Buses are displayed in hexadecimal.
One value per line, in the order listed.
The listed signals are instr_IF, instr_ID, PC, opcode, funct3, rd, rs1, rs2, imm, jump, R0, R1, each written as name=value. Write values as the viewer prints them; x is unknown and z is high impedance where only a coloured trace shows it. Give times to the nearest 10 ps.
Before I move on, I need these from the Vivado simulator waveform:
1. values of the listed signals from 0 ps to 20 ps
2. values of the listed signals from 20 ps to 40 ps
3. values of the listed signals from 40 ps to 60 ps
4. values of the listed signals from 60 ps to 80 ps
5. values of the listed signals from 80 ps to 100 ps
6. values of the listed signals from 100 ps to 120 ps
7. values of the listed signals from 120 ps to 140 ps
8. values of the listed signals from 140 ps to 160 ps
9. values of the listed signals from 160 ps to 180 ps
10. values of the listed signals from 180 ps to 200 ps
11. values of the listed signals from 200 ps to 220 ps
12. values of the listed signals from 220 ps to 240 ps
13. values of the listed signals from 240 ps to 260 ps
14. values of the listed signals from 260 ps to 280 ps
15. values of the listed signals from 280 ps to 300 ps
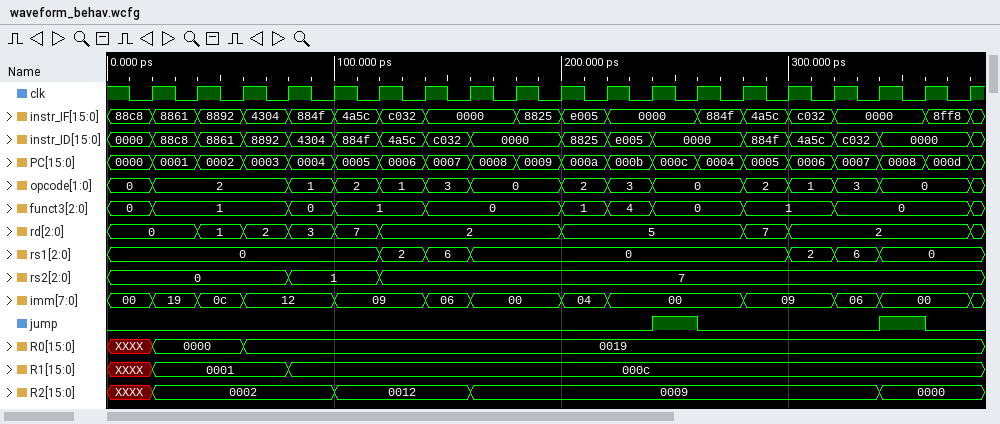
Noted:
instr_IF=88c8, instr_ID=0000, PC=0000, opcode=0, funct3=0, rd=0, rs1=0, rs2=0, imm=00, jump=0, R0=XXXX, R1=XXXX
instr_IF=8861, instr_ID=88c8, PC=0001, opcode=2, funct3=1, rd=0, rs1=0, rs2=0, imm=19, jump=0, R0=0000, R1=0001
instr_IF=8892, instr_ID=8861, PC=0002, opcode=2, funct3=1, rd=1, rs1=0, rs2=0, imm=0c, jump=0, R0=0000, R1=0001
instr_IF=4304, instr_ID=8892, PC=0003, opcode=2, funct3=1, rd=2, rs1=0, rs2=0, imm=12, jump=0, R0=0019, R1=0001
instr_IF=884f, instr_ID=4304, PC=0004, opcode=1, funct3=0, rd=3, rs1=0, rs2=1, imm=12, jump=0, R0=0019, R1=000c
instr_IF=4a5c, instr_ID=884f, PC=0005, opcode=2, funct3=1, rd=7, rs1=0, rs2=1, imm=09, jump=0, R0=0019, R1=000c
instr_IF=c032, instr_ID=4a5c, PC=0006, opcode=1, funct3=1, rd=2, rs1=2, rs2=7, imm=09, jump=0, R0=0019, R1=000c
instr_IF=0000, instr_ID=c032, PC=0007, opcode=3, funct3=0, rd=2, rs1=6, rs2=7, imm=06, jump=0, R0=0019, R1=000c
instr_IF=0000, instr_ID=0000, PC=0008, opcode=0, funct3=0, rd=2, rs1=0, rs2=7, imm=00, jump=0, R0=0019, R1=000c
instr_IF=8825, instr_ID=0000, PC=0009, opcode=0, funct3=0, rd=2, rs1=0, rs2=7, imm=00, jump=0, R0=0019, R1=000c
instr_IF=e005, instr_ID=8825, PC=000a, opcode=2, funct3=1, rd=5, rs1=0, rs2=7, imm=04, jump=0, R0=0019, R1=000c
instr_IF=0000, instr_ID=e005, PC=000b, opcode=3, funct3=4, rd=5, rs1=0, rs2=7, imm=00, jump=0, R0=0019, R1=000c
instr_IF=0000, instr_ID=0000, PC=000c, opcode=0, funct3=0, rd=5, rs1=0, rs2=7, imm=00, jump=1, R0=0019, R1=000c
instr_IF=884f, instr_ID=0000, PC=0004, opcode=0, funct3=0, rd=5, rs1=0, rs2=7, imm=00, jump=0, R0=0019, R1=000c
instr_IF=4a5c, instr_ID=884f, PC=0005, opcode=2, funct3=1, rd=7, rs1=0, rs2=7, imm=09, jump=0, R0=0019, R1=000c
